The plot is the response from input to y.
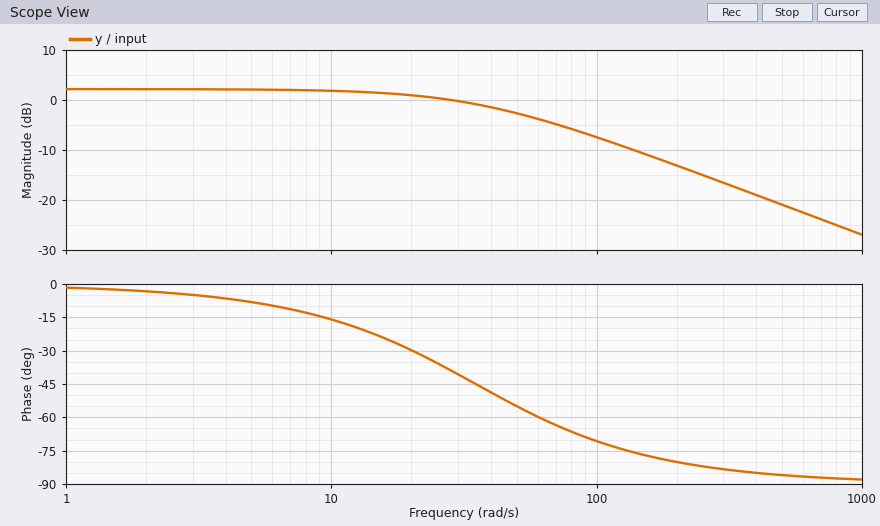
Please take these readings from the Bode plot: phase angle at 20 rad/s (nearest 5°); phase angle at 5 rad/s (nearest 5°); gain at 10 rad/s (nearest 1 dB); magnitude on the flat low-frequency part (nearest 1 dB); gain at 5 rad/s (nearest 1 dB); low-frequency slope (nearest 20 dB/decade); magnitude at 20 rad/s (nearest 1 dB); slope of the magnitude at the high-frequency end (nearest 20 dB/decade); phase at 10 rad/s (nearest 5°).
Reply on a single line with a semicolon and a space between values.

-30°; -10°; 2 dB; 2 dB; 2 dB; 0 dB/decade; 1 dB; -20 dB/decade; -15°
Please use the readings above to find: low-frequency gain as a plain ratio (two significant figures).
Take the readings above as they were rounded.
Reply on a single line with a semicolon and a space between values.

1.3
